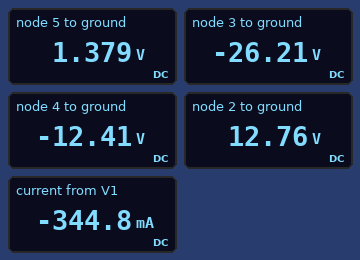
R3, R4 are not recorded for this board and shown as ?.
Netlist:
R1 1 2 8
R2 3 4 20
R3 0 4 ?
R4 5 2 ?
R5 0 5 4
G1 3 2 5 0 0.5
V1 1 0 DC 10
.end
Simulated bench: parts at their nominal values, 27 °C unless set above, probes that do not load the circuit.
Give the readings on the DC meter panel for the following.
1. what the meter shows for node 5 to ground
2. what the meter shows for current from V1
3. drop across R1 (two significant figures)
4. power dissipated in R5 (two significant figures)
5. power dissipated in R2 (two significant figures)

1.379 V
-344.8 mA
2.8 V
480 mW
9.5 W
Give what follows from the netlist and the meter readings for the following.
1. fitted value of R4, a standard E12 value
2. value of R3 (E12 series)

33 Ω
18 Ω
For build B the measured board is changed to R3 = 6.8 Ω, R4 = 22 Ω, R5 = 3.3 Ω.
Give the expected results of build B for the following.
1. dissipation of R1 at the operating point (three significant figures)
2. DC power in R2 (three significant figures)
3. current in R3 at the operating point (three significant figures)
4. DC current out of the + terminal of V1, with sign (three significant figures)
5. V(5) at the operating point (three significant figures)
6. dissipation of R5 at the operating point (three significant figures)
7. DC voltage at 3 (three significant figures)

837 mW
13.5 W
821 mA
-323 mA
1.64 V
817 mW
-22.0 V
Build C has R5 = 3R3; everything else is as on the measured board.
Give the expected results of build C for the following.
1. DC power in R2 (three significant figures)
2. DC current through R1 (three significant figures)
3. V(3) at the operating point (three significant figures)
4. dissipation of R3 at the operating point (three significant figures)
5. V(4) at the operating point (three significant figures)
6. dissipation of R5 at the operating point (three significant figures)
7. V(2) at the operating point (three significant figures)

5.63 W
209 mA
-20.2 V
5.07 W
-9.55 V
341 mW
11.7 V
